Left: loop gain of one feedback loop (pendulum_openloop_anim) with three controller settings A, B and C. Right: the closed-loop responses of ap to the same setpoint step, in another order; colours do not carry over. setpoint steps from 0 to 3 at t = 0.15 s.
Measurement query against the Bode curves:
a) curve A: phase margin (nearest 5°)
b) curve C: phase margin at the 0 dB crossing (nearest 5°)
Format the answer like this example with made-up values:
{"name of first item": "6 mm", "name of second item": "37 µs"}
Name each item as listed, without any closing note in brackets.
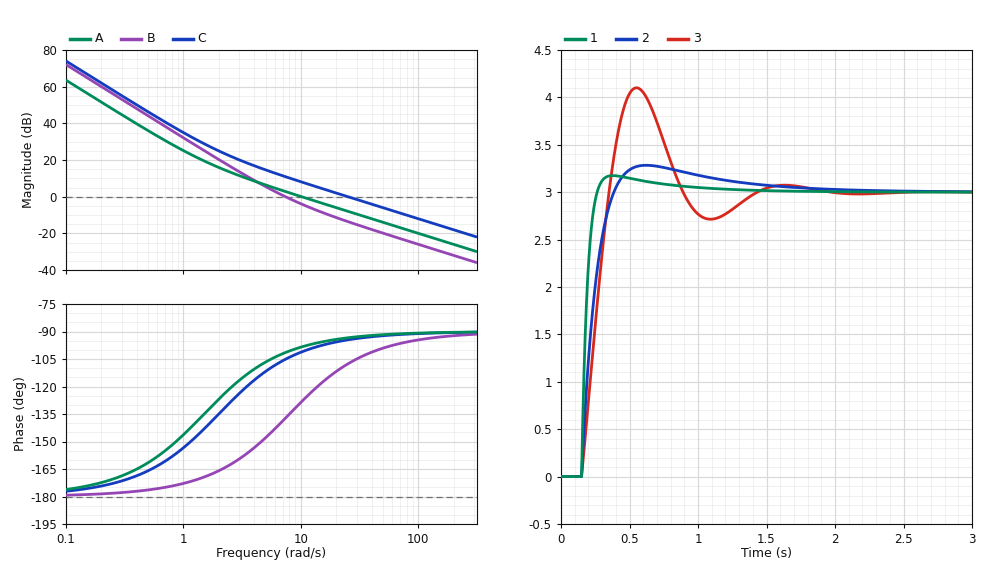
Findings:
{"curve A: phase margin": "80°", "curve C: phase margin at the 0 dB crossing": "85°"}
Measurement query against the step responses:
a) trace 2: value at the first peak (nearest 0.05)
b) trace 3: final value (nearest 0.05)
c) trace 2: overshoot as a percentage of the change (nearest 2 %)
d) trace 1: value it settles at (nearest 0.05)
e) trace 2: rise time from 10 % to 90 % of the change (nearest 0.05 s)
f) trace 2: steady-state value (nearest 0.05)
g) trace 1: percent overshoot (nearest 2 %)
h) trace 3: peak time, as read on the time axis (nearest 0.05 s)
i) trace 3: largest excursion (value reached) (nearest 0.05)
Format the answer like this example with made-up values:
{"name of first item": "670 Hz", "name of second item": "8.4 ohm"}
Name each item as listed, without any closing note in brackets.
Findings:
{"trace 2: value at the first peak": "3.30", "trace 3: final value": "3.00", "trace 2: overshoot as a percentage of the change": "10 %", "trace 1: value it settles at": "3.00", "trace 2: rise time from 10 % to 90 % of the change": "0.15 s", "trace 2: steady-state value": "3.00", "trace 1: percent overshoot": "6 %", "trace 3: peak time, as read on the time axis": "0.55 s", "trace 3: largest excursion (value reached)": "4.10"}
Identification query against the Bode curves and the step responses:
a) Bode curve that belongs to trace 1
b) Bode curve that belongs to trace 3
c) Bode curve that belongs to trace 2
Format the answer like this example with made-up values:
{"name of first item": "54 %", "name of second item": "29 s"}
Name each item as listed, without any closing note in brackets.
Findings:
{"Bode curve that belongs to trace 1": "C", "Bode curve that belongs to trace 3": "B", "Bode curve that belongs to trace 2": "A"}
